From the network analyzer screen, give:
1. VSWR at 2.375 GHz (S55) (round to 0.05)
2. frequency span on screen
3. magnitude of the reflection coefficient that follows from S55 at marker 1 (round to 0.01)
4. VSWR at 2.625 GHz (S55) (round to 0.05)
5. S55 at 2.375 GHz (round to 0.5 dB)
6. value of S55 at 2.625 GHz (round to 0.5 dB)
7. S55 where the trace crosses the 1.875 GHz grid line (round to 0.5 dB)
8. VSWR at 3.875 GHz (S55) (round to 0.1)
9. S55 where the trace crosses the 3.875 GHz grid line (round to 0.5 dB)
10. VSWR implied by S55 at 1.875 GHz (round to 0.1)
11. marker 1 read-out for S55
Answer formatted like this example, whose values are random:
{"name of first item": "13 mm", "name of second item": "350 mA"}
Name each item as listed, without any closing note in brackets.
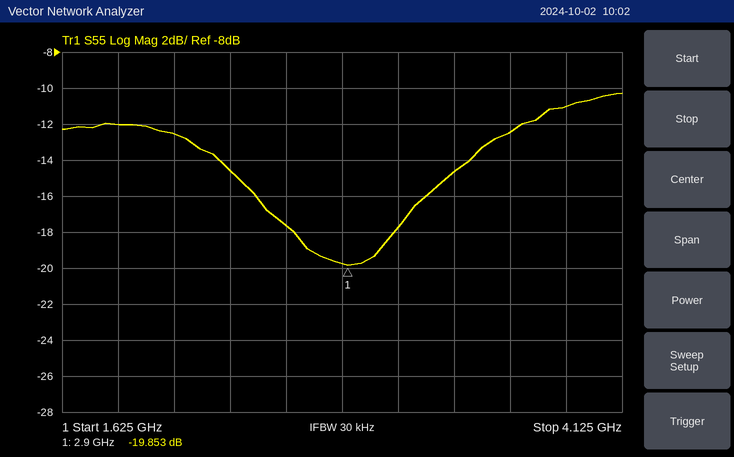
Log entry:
{"VSWR at 2.375 GHz (S55)": "1.45", "frequency span on screen": "2.5 GHz", "magnitude of the reflection coefficient that follows from S55 at marker 1": "0.10", "VSWR at 2.625 GHz (S55)": "1.30", "S55 at 2.375 GHz": "-14.5 dB", "value of S55 at 2.625 GHz": "-17.5 dB", "S55 where the trace crosses the 1.875 GHz grid line": "-12.0 dB", "VSWR at 3.875 GHz (S55)": "1.8", "S55 where the trace crosses the 3.875 GHz grid line": "-11.0 dB", "VSWR implied by S55 at 1.875 GHz": "1.7", "marker 1 read-out for S55": "-19.853 dB"}
